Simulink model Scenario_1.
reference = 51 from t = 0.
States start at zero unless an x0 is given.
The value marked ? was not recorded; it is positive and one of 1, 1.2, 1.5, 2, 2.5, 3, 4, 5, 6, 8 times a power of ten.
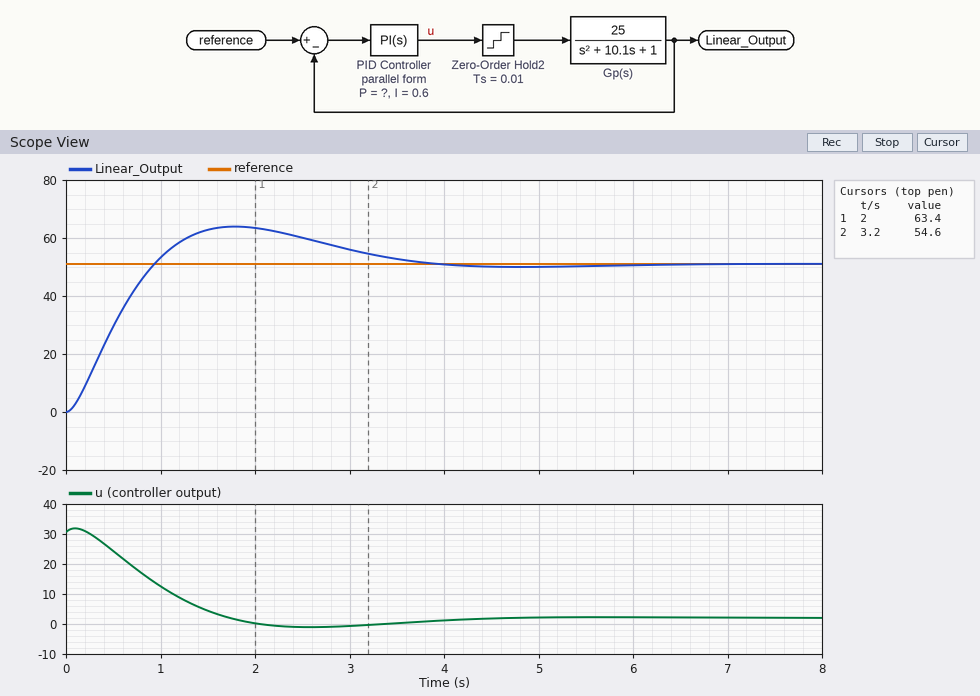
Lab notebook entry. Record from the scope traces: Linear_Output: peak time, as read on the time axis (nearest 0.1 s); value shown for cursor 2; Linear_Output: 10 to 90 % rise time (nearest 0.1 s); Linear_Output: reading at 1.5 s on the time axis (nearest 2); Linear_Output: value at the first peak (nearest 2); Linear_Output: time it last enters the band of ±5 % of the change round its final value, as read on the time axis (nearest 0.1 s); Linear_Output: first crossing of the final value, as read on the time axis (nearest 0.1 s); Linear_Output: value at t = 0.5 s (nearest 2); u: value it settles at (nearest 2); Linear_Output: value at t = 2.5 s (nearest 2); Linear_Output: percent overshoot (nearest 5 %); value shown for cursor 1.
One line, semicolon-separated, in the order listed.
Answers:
1.8 s; 54.6; 0.7 s; 62; 64; 3.4 s; 0.9 s; 30; 2; 60; 25 %; 63.4
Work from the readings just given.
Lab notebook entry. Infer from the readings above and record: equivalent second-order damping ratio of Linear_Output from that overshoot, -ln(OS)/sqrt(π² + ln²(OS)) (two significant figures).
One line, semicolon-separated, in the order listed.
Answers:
0.40
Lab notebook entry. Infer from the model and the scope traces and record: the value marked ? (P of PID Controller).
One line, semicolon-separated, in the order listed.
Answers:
0.6
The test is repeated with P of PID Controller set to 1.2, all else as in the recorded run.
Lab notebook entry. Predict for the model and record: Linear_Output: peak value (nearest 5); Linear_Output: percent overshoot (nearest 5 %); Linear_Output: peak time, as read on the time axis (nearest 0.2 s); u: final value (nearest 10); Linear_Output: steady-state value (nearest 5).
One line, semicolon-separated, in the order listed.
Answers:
55; 10 %; 1.2 s; 0; 50
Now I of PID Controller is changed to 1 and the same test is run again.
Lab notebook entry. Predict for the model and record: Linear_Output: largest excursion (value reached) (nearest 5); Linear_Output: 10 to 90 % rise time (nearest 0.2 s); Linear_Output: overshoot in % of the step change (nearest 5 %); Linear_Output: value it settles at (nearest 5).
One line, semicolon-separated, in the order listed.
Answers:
70; 0.6 s; 35 %; 50
